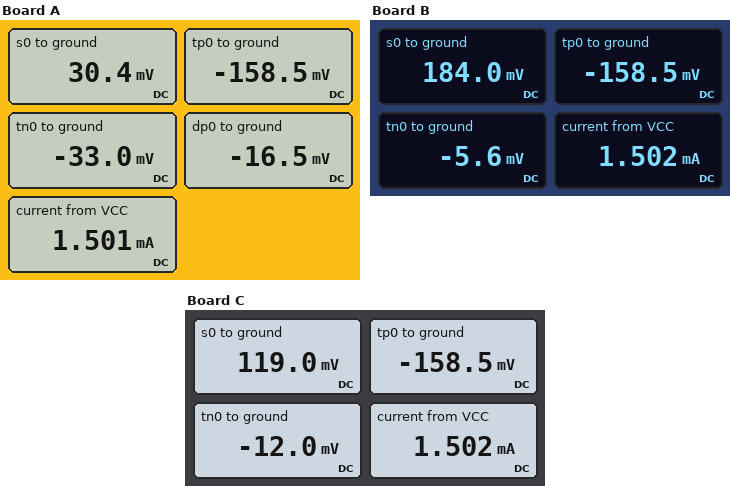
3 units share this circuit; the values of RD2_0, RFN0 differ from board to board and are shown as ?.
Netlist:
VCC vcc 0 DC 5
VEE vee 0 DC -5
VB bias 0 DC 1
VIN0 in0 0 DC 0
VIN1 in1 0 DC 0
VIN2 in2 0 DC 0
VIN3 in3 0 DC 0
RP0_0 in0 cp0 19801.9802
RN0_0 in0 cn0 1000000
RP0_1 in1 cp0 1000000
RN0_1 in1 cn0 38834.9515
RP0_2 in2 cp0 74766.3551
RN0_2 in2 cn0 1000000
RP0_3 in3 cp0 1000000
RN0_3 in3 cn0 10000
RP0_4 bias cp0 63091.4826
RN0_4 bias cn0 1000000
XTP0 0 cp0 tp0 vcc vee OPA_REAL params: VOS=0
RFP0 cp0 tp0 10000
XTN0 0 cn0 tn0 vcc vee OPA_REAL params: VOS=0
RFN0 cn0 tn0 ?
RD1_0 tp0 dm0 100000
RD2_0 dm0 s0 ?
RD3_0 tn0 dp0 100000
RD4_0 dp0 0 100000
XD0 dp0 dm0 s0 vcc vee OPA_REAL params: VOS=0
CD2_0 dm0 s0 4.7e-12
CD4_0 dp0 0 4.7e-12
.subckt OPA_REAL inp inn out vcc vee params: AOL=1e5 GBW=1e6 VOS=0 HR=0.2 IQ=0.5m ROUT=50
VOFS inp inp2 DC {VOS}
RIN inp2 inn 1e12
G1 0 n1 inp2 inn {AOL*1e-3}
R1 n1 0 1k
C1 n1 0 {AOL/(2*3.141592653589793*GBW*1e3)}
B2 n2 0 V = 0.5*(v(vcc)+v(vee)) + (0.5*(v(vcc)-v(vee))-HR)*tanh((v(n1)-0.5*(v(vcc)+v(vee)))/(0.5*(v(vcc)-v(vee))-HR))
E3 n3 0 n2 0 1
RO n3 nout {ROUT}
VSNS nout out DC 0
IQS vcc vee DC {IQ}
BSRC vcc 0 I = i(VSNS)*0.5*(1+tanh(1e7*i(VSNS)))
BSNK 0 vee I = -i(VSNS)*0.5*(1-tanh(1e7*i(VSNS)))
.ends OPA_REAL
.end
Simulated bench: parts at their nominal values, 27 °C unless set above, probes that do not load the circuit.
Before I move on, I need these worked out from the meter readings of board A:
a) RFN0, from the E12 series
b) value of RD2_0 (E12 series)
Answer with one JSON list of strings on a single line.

["33 kΩ", "33 kΩ"]
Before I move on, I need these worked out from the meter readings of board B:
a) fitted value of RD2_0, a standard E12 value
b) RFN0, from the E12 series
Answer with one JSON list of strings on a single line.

["120 kΩ", "5.6 kΩ"]
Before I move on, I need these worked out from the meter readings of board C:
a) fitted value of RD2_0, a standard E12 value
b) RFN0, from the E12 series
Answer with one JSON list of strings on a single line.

["82 kΩ", "12 kΩ"]
